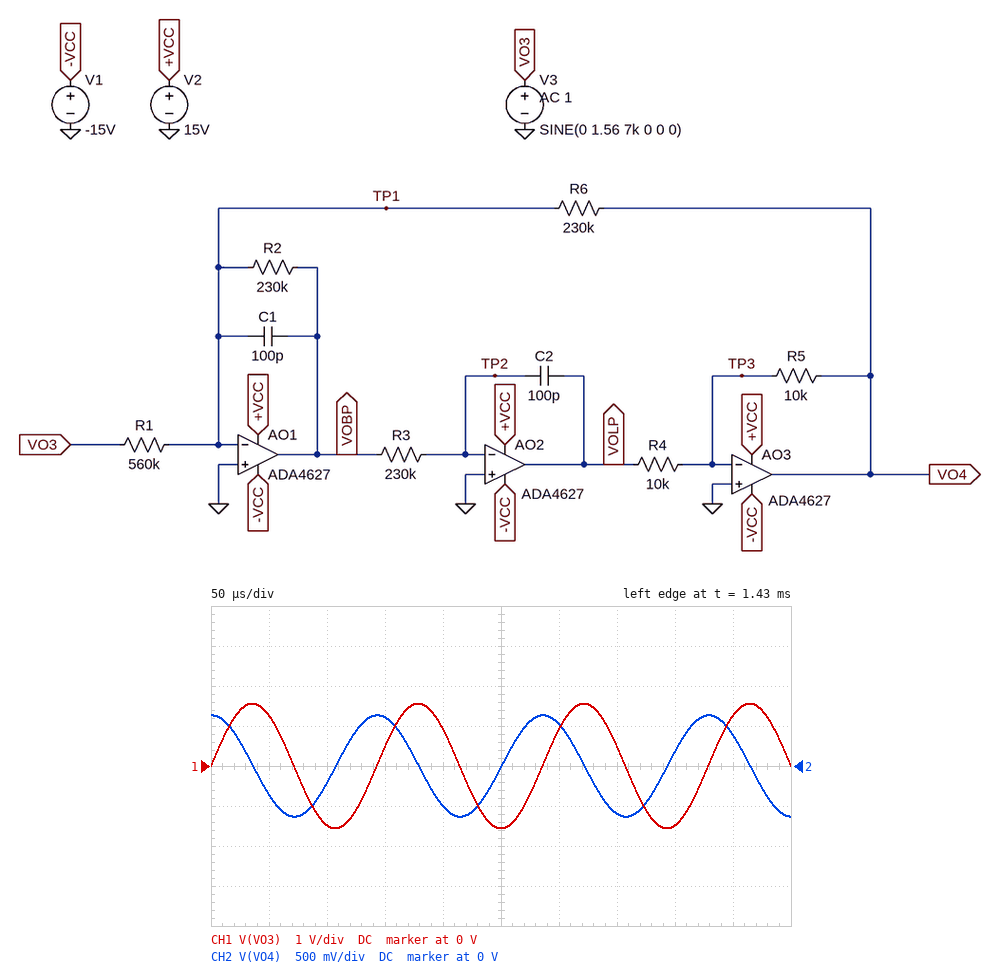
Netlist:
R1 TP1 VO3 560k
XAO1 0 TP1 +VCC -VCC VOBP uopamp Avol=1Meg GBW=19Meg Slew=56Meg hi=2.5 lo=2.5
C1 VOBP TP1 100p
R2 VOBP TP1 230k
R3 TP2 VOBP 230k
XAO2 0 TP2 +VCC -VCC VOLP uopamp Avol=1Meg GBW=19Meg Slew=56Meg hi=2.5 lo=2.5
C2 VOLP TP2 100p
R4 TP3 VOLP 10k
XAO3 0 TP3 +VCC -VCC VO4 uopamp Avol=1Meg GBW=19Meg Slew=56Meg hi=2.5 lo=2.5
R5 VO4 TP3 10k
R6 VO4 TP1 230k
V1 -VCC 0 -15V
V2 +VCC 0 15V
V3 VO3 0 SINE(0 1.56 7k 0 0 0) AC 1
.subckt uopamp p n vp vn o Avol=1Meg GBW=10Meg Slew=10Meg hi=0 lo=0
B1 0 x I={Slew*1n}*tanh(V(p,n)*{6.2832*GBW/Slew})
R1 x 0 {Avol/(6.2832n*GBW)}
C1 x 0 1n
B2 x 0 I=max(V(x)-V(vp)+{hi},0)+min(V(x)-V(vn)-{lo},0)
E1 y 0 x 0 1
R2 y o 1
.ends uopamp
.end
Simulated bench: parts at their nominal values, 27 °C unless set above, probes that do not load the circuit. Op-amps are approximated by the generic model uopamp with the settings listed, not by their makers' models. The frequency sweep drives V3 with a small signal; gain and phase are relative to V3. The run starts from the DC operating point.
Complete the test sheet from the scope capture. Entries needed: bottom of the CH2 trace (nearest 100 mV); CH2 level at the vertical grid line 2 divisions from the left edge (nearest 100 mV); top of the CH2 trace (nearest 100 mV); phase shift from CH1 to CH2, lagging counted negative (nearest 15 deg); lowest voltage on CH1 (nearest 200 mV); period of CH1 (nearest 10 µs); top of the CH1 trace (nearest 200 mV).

-600 mV
-200 mV
600 mV
90 deg
-1.6 V
140 µs
1.6 V
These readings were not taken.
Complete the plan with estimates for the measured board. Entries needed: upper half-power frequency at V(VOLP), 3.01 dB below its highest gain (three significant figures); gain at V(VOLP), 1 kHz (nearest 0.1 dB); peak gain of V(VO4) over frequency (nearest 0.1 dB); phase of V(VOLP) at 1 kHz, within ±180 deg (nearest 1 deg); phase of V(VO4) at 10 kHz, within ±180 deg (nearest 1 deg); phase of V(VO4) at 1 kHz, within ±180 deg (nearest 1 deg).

8.09 kHz
-7.6 dB
-6.5 dB
-8 deg
53 deg
172 deg
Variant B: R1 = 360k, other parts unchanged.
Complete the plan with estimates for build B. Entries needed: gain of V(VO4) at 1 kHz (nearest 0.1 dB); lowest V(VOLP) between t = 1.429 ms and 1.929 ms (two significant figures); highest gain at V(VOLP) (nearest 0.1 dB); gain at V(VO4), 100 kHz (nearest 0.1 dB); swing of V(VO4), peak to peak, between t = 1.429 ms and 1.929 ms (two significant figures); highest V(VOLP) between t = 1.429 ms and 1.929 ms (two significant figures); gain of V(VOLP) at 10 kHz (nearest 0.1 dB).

-3.8 dB
-990 mV
-2.6 dB
-50.3 dB
2.0 V
990 mV
-9.0 dB
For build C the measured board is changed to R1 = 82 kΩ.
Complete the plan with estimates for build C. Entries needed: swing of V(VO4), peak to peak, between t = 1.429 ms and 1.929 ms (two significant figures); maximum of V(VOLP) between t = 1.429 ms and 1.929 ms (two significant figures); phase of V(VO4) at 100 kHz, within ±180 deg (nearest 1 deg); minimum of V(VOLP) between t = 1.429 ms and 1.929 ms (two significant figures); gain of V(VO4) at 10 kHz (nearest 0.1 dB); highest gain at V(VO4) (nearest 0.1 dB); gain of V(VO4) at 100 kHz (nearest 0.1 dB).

8.7 V
4.3 V
3 deg
-4.3 V
3.8 dB
10.2 dB
-37.4 dB
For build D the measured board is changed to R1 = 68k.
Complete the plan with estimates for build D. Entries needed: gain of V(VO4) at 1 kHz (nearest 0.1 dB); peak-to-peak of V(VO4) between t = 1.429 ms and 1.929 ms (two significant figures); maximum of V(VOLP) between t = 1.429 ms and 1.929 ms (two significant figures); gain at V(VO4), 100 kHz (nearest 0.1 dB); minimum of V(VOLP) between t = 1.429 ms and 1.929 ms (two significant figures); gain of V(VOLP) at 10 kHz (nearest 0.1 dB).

10.7 dB
10 V
5.2 V
-35.8 dB
-5.2 V
5.4 dB
